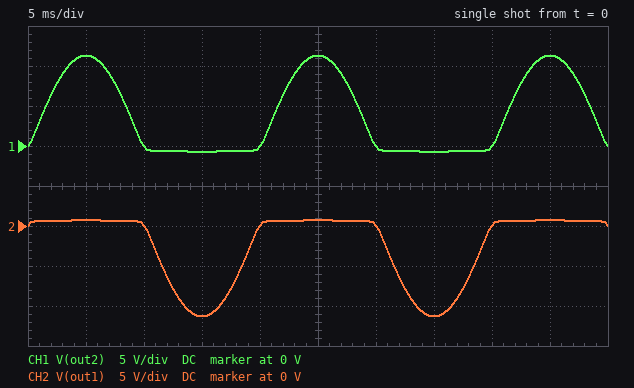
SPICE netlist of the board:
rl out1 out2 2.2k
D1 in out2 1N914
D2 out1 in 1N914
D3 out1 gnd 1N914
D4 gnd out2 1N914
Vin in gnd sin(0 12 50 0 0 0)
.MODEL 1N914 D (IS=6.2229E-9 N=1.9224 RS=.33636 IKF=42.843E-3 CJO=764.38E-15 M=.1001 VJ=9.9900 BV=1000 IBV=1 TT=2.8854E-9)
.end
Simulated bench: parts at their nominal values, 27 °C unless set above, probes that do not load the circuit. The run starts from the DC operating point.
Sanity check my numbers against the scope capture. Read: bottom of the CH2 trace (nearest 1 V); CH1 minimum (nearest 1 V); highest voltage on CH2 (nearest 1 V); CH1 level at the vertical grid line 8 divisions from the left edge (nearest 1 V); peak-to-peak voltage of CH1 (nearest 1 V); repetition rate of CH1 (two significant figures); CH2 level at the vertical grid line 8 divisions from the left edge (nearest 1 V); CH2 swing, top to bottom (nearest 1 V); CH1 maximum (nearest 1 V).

-11 V
-1 V
1 V
0 V
12 V
50 Hz
0 V
12 V
11 V
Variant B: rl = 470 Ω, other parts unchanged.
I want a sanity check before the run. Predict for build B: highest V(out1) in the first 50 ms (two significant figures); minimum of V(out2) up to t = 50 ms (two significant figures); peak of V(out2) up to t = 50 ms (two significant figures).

790 mV
-790 mV
11 V
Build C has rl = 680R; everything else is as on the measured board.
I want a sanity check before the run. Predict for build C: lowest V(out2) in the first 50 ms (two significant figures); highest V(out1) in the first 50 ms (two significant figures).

-770 mV
770 mV
